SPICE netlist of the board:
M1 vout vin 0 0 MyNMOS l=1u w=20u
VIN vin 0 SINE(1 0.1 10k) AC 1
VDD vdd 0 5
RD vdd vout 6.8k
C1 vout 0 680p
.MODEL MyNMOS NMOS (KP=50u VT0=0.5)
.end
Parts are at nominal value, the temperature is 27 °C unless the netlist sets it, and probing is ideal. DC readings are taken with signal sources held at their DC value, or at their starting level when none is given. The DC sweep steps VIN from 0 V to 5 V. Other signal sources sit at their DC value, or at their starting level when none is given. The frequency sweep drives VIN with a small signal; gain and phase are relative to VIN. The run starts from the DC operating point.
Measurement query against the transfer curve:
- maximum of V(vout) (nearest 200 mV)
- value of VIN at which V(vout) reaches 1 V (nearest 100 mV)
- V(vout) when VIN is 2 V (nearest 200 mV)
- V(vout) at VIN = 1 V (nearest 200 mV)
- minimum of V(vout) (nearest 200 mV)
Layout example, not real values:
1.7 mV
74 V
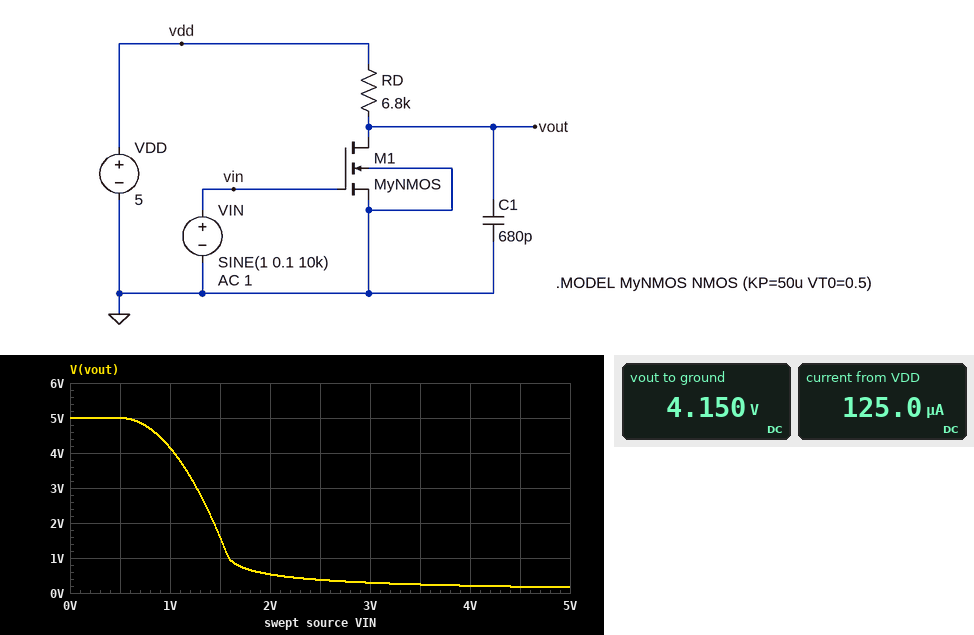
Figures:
5.0 V
1.6 V
600 mV
4.2 V
200 mV
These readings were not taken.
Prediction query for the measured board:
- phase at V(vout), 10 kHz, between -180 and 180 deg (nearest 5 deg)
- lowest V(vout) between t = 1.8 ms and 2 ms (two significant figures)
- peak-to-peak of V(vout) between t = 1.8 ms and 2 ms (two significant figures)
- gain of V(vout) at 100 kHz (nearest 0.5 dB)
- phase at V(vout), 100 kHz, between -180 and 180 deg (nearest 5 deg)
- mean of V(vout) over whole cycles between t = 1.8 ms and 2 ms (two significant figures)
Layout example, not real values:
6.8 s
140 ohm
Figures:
165 deg
3.8 V
650 mV
1.0 dB
110 deg
4.1 V
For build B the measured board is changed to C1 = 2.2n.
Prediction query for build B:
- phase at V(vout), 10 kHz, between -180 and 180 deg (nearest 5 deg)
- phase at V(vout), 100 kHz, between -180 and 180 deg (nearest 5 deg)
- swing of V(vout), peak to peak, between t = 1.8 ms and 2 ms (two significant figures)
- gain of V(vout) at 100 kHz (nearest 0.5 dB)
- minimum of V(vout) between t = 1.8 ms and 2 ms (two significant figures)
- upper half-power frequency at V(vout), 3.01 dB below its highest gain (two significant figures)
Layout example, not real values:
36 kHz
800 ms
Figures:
135 deg
95 deg
500 mV
-9.0 dB
3.9 V
11 kHz
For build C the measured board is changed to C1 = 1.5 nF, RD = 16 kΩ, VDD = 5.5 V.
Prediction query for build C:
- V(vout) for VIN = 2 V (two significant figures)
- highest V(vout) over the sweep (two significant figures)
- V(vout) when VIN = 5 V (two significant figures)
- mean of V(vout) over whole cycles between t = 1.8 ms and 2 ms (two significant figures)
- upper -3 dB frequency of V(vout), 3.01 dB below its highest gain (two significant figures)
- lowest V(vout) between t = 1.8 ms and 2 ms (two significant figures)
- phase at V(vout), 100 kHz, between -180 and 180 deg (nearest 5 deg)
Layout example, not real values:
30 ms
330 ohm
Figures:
240 mV
5.5 V
76 mV
3.5 V
6.6 kHz
3.0 V
95 deg
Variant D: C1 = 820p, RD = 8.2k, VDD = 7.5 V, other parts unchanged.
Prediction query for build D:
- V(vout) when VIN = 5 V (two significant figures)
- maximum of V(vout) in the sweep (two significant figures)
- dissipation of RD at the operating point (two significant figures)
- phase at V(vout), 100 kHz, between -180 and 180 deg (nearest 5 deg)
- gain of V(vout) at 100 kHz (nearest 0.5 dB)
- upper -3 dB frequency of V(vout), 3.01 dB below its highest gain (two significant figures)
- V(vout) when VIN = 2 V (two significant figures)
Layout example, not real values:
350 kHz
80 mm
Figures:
200 mV
7.5 V
130 µW
105 deg
-0.5 dB
24 kHz
730 mV
